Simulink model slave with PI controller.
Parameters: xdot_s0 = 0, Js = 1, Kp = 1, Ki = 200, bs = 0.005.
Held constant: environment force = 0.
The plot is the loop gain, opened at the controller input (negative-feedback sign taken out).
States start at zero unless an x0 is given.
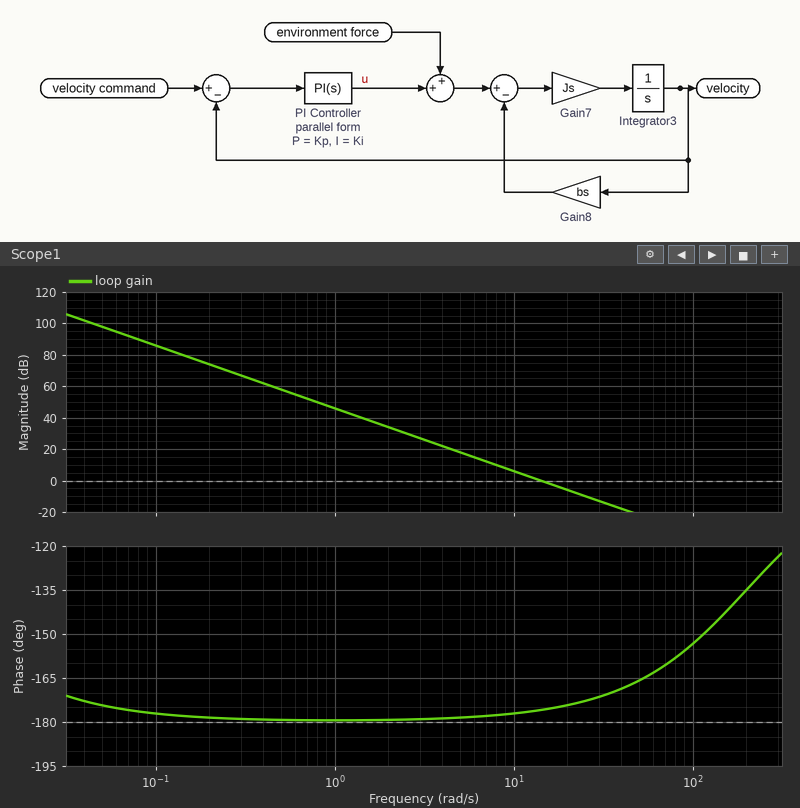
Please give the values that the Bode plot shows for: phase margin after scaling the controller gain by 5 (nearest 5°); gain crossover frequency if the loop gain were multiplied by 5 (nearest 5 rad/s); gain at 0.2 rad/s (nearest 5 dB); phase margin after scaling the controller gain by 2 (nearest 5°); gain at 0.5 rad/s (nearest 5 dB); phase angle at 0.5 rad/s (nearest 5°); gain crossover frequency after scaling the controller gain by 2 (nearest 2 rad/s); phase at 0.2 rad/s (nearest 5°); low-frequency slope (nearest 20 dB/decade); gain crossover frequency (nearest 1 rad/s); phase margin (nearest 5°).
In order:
10°
30 rad/s
75 dB
5°
60 dB
-180°
20 rad/s
-180°
-40 dB/decade
14 rad/s
5°
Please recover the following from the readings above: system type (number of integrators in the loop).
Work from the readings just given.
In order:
2
